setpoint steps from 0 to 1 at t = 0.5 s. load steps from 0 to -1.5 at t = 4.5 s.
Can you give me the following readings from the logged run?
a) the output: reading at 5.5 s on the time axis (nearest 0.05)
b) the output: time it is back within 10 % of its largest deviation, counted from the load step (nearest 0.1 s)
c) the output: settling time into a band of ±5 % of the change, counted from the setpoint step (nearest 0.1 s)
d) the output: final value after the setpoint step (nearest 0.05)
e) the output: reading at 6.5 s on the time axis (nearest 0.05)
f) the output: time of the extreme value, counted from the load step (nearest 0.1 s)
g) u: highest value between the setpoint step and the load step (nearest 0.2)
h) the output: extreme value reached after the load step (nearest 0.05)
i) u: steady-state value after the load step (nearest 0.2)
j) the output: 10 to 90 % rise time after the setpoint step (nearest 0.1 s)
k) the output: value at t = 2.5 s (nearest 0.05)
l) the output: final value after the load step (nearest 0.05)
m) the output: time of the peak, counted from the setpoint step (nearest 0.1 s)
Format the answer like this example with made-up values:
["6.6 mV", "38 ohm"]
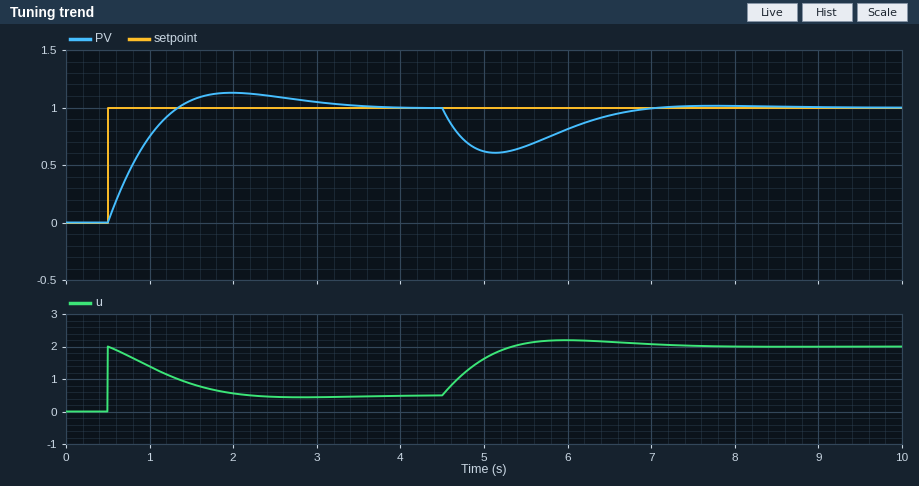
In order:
["0.65", "2.2 s", "2.5 s", "1.00", "0.95", "0.6 s", "2.0", "0.60", "2.0", "0.6 s", "1.10", "1.00", "1.5 s"]
